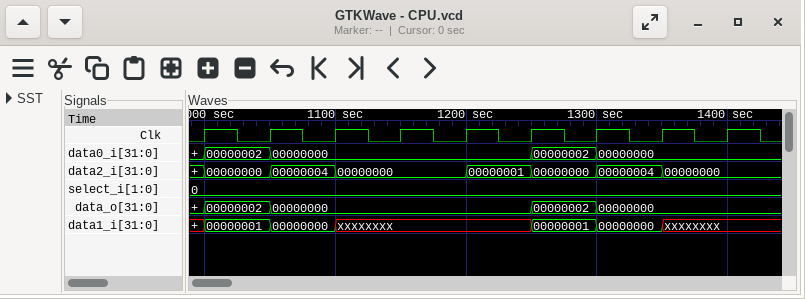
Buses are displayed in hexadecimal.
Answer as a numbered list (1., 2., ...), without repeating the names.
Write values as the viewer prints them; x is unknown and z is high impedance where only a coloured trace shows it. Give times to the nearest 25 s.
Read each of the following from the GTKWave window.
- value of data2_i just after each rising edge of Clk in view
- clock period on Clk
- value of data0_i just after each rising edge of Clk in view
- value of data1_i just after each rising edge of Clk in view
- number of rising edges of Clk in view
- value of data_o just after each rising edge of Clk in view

1. 00000000, 00000004, 00000000, 00000000, 00000001, 00000000, 00000004, 00000000, 00000000
2. 50 s
3. 00000002, 00000000, 00000000, 00000000, 00000000, 00000002, 00000000, 00000000, 00000000
4. 00000001, 00000000, xxxxxxxx, xxxxxxxx, xxxxxxxx, 00000001, 00000000, xxxxxxxx, xxxxxxxx
5. 9
6. 00000002, 00000000, 00000000, 00000000, 00000000, 00000002, 00000000, 00000000, 00000000
